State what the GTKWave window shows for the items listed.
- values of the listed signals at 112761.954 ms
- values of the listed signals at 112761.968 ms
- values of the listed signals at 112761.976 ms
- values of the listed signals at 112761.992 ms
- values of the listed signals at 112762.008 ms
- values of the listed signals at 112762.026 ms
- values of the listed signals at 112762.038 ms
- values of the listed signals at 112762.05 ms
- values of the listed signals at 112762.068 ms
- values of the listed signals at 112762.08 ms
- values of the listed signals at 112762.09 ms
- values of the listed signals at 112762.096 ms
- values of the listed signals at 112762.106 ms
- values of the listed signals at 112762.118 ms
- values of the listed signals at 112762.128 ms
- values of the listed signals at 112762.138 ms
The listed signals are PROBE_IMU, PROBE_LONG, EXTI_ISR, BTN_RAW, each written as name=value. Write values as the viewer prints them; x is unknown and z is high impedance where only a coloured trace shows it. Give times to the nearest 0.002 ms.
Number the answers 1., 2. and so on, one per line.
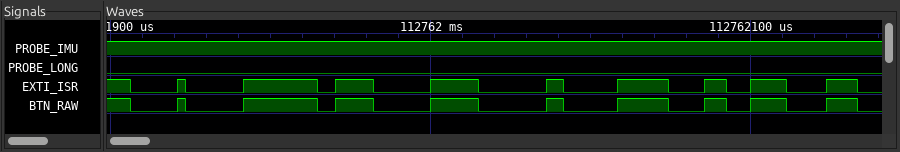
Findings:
1. PROBE_IMU=1, PROBE_LONG=0, EXTI_ISR=1, BTN_RAW=1
2. PROBE_IMU=1, PROBE_LONG=0, EXTI_ISR=0, BTN_RAW=0
3. PROBE_IMU=1, PROBE_LONG=0, EXTI_ISR=1, BTN_RAW=1
4. PROBE_IMU=1, PROBE_LONG=0, EXTI_ISR=0, BTN_RAW=0
5. PROBE_IMU=1, PROBE_LONG=0, EXTI_ISR=1, BTN_RAW=1
6. PROBE_IMU=1, PROBE_LONG=0, EXTI_ISR=0, BTN_RAW=0
7. PROBE_IMU=1, PROBE_LONG=0, EXTI_ISR=1, BTN_RAW=1
8. PROBE_IMU=1, PROBE_LONG=0, EXTI_ISR=0, BTN_RAW=0
9. PROBE_IMU=1, PROBE_LONG=0, EXTI_ISR=1, BTN_RAW=1
10. PROBE_IMU=1, PROBE_LONG=0, EXTI_ISR=0, BTN_RAW=0
11. PROBE_IMU=1, PROBE_LONG=0, EXTI_ISR=1, BTN_RAW=1
12. PROBE_IMU=1, PROBE_LONG=0, EXTI_ISR=0, BTN_RAW=0
13. PROBE_IMU=1, PROBE_LONG=0, EXTI_ISR=1, BTN_RAW=1
14. PROBE_IMU=1, PROBE_LONG=0, EXTI_ISR=0, BTN_RAW=0
15. PROBE_IMU=1, PROBE_LONG=0, EXTI_ISR=1, BTN_RAW=1
16. PROBE_IMU=1, PROBE_LONG=0, EXTI_ISR=0, BTN_RAW=0
